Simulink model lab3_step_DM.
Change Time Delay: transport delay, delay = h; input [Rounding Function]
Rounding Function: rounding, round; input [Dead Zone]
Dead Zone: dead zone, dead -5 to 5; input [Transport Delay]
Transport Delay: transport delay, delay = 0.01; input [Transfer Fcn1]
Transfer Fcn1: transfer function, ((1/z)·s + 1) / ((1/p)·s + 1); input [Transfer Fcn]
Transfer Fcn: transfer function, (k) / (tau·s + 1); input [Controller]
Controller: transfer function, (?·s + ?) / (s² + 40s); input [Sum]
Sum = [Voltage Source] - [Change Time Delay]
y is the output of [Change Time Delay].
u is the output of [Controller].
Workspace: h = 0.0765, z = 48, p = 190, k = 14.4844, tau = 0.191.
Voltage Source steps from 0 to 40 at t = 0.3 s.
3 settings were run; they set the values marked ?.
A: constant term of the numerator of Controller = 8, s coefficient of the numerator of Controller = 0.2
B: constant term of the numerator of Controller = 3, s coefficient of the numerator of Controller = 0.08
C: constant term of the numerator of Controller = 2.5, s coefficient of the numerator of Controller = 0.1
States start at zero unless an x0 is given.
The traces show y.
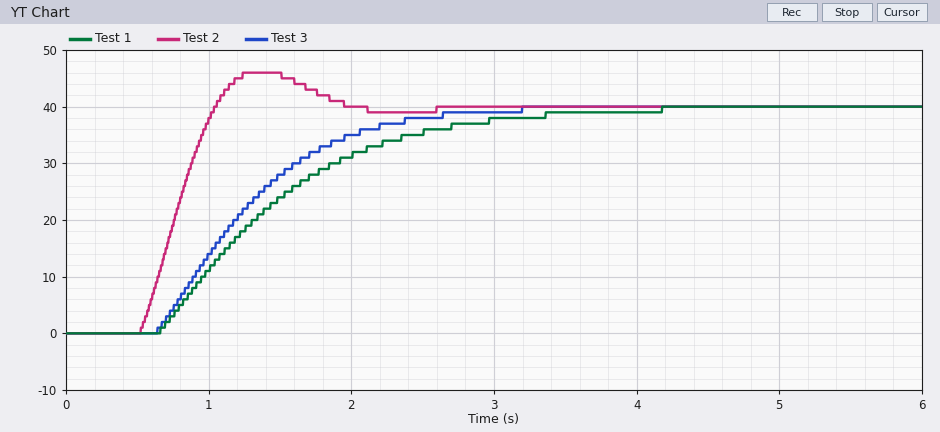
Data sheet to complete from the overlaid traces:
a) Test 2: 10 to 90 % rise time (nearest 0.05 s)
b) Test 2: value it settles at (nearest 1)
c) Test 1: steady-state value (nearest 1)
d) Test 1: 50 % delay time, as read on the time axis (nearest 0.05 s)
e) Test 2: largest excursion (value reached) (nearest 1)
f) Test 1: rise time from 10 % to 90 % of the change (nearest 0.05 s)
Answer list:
0.40 s
40
40
1.30 s
46
1.75 s
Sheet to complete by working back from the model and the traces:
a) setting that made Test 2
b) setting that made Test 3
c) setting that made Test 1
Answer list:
A
B
C
